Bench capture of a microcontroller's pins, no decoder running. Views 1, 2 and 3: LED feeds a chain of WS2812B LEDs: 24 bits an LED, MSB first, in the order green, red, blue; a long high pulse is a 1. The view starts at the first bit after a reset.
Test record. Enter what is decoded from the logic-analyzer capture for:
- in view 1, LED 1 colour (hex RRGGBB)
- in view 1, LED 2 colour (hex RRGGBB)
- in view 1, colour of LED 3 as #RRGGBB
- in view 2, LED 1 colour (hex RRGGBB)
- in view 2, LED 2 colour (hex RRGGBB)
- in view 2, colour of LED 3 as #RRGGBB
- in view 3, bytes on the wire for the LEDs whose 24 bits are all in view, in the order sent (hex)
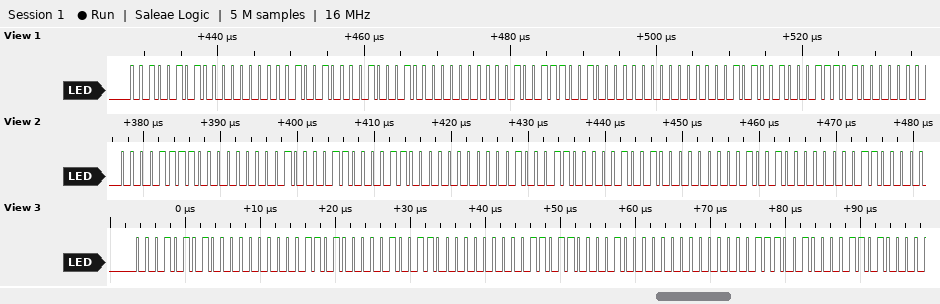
#002524
#002227
#002029
#000F43
#000C46
#000948
15 00 34 13 00 36 10 00 39
